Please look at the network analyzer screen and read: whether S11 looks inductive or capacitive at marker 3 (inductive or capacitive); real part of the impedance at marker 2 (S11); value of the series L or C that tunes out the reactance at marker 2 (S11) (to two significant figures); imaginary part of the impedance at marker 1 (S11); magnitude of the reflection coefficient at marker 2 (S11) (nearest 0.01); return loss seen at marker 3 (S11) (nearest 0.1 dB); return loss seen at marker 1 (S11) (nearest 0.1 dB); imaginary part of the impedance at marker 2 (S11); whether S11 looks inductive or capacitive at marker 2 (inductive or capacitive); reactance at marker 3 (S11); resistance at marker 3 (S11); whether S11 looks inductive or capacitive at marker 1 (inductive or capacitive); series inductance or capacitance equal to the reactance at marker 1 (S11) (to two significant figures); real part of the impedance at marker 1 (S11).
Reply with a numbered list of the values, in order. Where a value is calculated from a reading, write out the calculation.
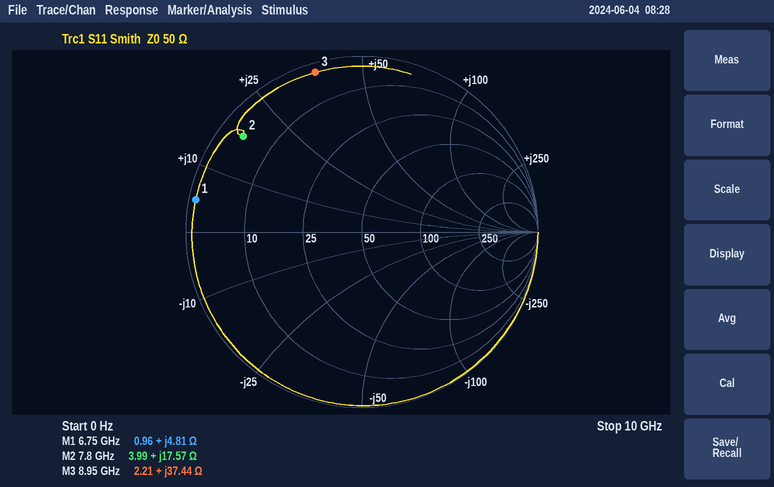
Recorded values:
1. inductive
2. 3.99 Ω
3. C = 1/(2π × 7.8 GHz × 17.57 Ω) ≈ 1.2 pF
4. +4.81 Ω
5. 0.87
6. 0.5 dB
7. 0.3 dB
8. +17.57 Ω
9. inductive
10. +37.44 Ω
11. 2.21 Ω
12. inductive
13. L = 4.81 Ω/(2π × 6.75 GHz) ≈ 113 pH, so 110 pH to two significant figures
14. 0.96 Ω
